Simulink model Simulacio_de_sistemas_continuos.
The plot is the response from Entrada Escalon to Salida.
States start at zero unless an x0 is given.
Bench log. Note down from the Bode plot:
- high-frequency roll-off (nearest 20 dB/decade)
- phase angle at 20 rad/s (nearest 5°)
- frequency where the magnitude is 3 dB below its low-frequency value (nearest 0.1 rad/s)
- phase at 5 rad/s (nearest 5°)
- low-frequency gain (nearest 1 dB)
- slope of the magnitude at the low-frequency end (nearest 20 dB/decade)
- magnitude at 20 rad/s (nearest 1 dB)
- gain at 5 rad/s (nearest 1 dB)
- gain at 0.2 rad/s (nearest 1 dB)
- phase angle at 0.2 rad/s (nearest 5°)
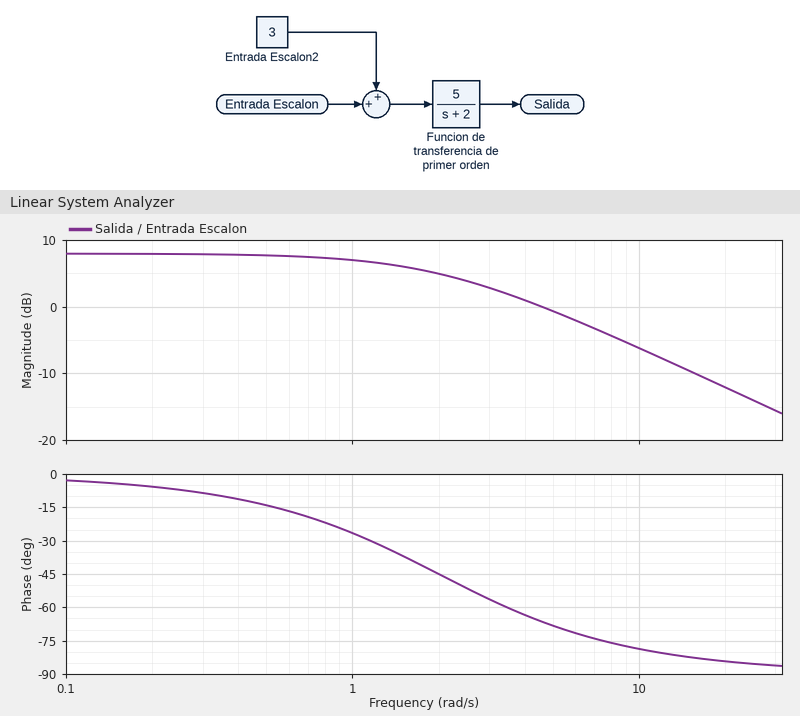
-20 dB/decade
-85°
2.0 rad/s
-70°
8 dB
0 dB/decade
-12 dB
-1 dB
8 dB
-5°
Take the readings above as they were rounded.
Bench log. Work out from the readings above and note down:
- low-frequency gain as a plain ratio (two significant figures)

2.5
